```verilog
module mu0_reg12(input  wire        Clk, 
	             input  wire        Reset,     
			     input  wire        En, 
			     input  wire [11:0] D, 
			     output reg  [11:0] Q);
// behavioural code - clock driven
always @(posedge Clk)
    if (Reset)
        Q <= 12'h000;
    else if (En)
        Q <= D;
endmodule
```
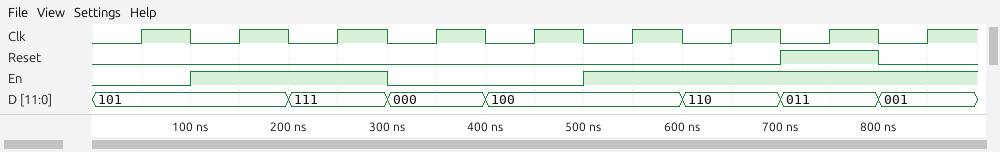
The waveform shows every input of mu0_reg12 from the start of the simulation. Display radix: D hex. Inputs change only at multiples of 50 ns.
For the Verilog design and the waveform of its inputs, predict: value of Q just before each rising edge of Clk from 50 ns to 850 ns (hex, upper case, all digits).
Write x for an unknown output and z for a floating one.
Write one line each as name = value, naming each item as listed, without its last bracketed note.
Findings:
value of Q just before each rising edge of Clk from 50 ns to 850 ns = x, x, 101, 111, 111, 111, 100, 110, 000
